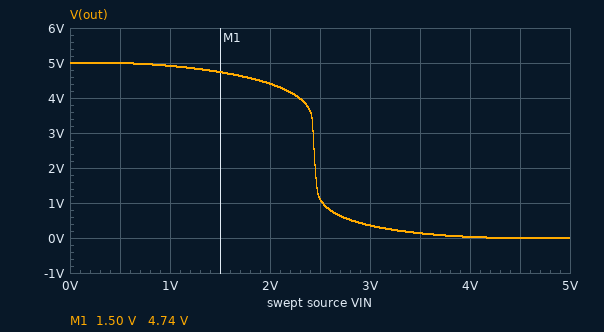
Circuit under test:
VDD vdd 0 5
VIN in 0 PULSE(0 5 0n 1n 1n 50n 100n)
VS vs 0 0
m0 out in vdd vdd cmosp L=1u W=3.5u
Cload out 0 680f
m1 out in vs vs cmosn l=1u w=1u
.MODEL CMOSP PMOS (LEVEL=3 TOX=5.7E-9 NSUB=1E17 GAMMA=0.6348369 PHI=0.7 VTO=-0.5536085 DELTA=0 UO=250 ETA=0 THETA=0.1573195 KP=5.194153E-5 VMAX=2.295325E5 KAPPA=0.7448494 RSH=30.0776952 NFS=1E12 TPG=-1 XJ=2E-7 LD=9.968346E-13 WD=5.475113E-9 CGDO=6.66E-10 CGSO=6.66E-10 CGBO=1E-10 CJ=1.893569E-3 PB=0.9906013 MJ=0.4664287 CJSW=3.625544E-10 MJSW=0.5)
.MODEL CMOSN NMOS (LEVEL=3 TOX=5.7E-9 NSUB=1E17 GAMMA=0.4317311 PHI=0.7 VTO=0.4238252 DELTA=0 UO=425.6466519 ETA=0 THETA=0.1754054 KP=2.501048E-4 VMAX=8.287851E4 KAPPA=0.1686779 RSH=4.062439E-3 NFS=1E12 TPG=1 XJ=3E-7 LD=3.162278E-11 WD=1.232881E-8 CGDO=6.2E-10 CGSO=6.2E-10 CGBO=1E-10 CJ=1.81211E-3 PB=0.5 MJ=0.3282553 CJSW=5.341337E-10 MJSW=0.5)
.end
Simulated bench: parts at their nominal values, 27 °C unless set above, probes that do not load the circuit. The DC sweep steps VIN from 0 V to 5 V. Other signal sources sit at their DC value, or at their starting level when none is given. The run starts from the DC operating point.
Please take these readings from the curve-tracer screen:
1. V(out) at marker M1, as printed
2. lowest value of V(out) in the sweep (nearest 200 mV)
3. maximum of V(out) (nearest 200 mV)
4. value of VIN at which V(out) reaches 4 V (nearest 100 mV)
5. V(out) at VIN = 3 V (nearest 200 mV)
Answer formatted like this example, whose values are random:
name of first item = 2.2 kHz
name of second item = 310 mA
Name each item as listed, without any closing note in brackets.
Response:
V(out) at marker M1, as printed = 4.74 V
lowest value of V(out) in the sweep = 0 V
maximum of V(out) = 5.0 V
value of VIN at which V(out) reaches 4 V = 2.3 V
V(out) at VIN = 3 V = 400 mV
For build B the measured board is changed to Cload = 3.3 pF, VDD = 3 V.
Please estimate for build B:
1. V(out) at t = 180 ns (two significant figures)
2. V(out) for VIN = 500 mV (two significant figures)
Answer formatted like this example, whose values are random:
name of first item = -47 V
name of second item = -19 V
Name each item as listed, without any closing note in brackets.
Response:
V(out) at t = 180 ns = 2.3 V
V(out) for VIN = 500 mV = 3.0 V
